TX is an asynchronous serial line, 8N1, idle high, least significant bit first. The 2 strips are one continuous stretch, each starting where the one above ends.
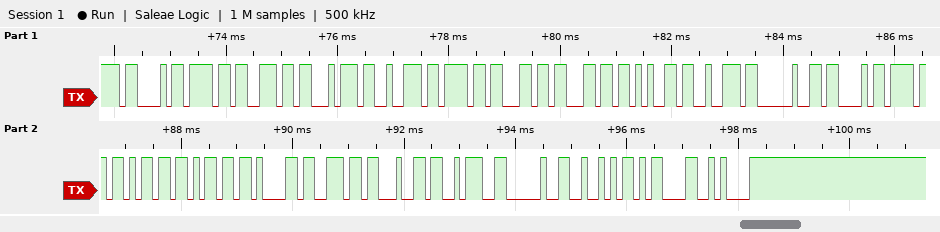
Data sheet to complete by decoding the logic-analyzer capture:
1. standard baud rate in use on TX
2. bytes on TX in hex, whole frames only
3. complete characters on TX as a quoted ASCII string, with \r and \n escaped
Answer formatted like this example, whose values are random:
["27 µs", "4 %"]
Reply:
["9600 baud", "43 6F 6E 74 72 6F 6C 6C 65 72 20 43 6F 6D 6D 61 6E 64 3A 20 52 0D 0A", "\"Controller Command: R\\r\\n\""]
